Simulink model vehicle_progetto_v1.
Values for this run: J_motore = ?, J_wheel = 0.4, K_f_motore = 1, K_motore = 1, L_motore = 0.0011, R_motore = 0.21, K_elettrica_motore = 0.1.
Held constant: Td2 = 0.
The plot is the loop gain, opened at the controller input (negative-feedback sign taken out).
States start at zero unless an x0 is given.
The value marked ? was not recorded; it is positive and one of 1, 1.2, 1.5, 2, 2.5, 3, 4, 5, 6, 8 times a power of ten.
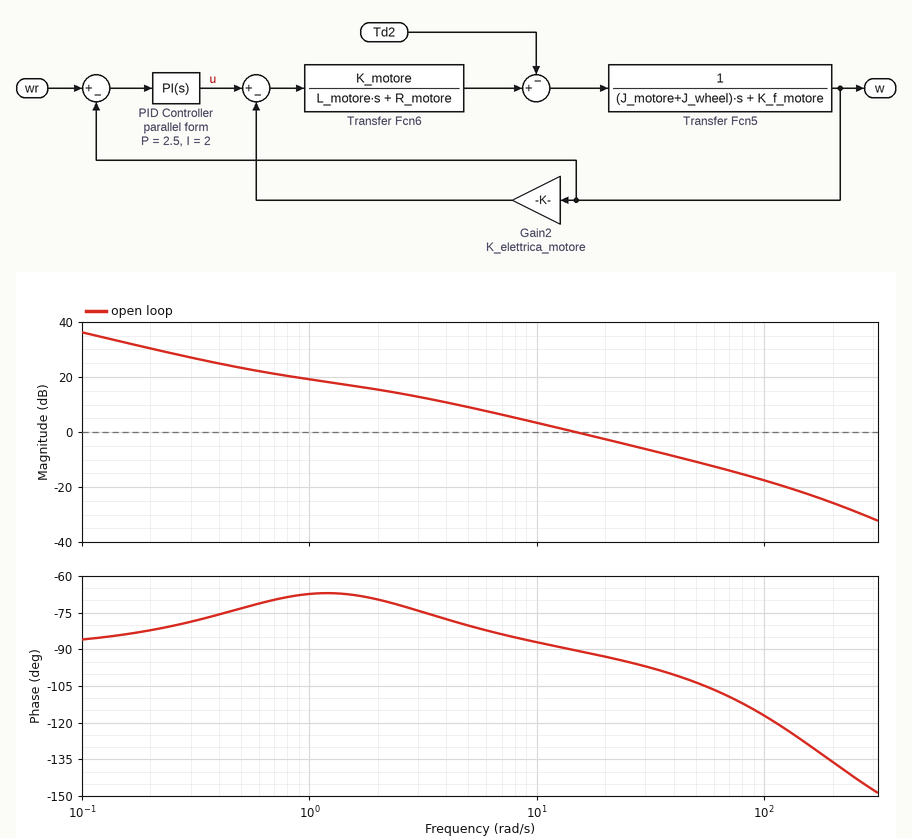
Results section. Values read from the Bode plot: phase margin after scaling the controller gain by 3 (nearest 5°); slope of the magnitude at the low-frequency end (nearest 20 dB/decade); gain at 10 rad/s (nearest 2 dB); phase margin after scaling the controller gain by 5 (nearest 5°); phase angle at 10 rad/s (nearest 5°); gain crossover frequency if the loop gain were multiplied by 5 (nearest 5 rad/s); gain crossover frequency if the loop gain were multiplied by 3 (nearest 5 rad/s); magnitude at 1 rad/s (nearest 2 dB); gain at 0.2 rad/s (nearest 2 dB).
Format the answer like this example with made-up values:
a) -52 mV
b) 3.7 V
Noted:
a) 80°
b) -20 dB/decade
c) 4 dB
d) 70°
e) -85°
f) 70 rad/s
g) 45 rad/s
h) 20 dB
i) 30 dB
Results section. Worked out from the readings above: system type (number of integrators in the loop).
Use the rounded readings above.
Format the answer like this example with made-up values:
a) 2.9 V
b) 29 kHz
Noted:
a) 1
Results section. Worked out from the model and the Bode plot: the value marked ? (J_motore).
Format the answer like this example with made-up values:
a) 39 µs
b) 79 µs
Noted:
a) 0.4
